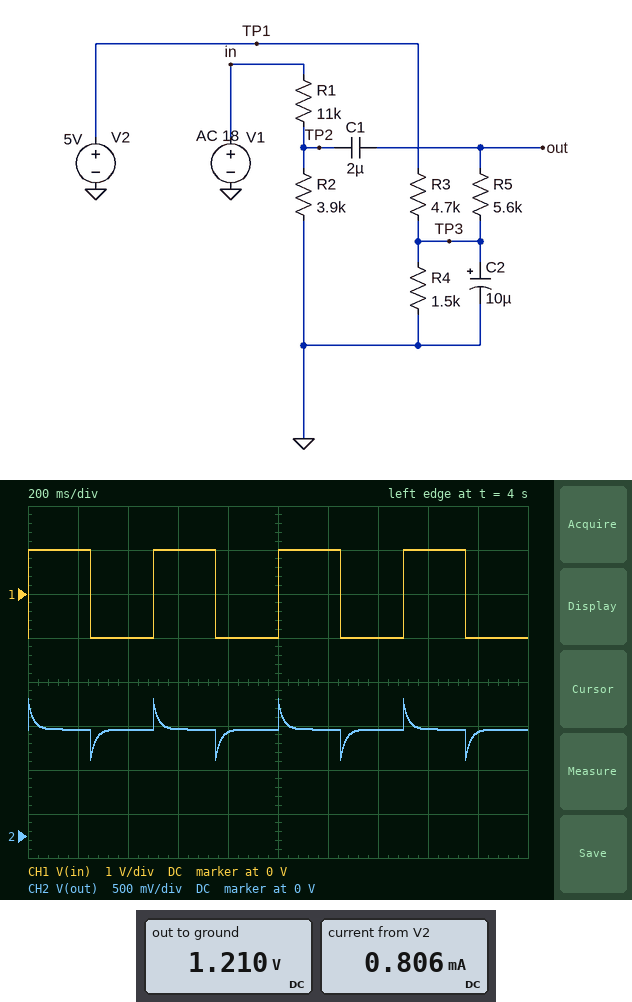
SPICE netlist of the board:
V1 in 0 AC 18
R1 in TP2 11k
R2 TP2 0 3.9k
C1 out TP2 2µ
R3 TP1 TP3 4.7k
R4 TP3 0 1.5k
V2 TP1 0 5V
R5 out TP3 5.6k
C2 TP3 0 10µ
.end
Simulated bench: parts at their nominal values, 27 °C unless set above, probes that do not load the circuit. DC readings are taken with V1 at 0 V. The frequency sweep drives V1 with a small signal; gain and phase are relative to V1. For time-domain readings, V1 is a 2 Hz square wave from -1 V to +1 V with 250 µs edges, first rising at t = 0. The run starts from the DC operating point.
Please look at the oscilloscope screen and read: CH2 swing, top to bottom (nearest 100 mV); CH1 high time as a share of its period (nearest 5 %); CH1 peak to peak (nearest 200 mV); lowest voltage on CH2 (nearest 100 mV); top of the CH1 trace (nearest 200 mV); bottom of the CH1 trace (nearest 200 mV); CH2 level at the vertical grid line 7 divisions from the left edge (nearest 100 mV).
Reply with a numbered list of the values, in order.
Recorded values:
1. 700 mV
2. 50 %
3. 2.0 V
4. 900 mV
5. 1.0 V
6. -1.0 V
7. 1.2 V
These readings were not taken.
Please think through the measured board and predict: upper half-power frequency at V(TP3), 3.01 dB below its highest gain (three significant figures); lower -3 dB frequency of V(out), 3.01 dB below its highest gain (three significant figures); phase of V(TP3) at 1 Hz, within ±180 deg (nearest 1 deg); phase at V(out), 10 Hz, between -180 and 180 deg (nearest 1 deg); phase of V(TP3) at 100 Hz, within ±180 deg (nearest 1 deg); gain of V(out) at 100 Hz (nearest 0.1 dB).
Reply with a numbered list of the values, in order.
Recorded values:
1. 29.7 Hz
2. 8.17 Hz
3. 79 deg
4. 38 deg
5. -76 deg
6. -15.3 dB
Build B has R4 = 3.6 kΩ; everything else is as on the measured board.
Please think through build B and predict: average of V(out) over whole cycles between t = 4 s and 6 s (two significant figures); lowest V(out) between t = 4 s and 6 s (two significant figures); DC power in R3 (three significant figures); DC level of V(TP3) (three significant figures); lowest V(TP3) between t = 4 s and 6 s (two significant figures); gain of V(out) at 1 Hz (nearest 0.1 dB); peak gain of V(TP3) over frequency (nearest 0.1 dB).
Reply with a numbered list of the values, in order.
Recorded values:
1. 2.2 V
2. 1.8 V
3. 1.71 mW
4. 2.17 V
5. 2.1 V
6. -32.1 dB
7. -31.8 dB
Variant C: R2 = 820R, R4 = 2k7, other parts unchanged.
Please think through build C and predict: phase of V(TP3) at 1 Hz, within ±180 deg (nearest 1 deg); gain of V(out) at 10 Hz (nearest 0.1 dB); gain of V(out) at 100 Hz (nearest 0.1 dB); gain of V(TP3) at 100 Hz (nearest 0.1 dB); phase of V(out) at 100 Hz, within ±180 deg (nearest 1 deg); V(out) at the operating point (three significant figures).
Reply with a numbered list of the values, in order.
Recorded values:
1. 78 deg
2. -28.1 dB
3. -24.4 dB
4. -55.4 dB
5. 7 deg
6. 1.82 V
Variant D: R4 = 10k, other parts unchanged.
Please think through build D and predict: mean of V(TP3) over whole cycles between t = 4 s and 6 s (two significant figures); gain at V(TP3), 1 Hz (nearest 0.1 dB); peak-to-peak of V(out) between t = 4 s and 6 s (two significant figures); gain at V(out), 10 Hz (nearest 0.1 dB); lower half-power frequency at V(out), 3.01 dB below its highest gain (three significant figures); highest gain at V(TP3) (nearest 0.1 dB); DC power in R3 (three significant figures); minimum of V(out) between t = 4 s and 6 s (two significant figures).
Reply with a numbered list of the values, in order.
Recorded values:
1. 3.4 V
2. -39.9 dB
3. 690 mV
4. -17.8 dB
5. 8.75 Hz
6. -30.4 dB
7. 544 µW
8. 3.1 V
